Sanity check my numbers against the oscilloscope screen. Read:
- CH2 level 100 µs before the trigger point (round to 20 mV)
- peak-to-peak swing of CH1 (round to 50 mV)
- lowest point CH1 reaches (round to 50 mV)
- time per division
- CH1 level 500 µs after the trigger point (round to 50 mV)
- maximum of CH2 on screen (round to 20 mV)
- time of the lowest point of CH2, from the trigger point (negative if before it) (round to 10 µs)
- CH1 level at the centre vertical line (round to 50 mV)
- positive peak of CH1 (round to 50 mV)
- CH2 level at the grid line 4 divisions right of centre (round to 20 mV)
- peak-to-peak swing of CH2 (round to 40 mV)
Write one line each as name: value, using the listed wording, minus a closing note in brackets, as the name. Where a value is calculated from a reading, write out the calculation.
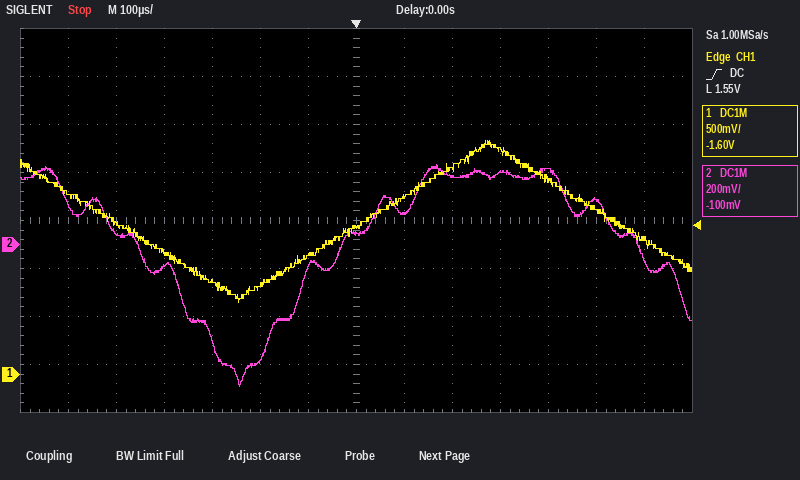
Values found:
CH2 level 100 µs before the trigger point: -100 mV
peak-to-peak swing of CH1: 2.45 V − (750 mV) = 1.70 V
lowest point CH1 reaches: 750 mV
time per division: 100 µs
CH1 level 500 µs after the trigger point: 1.70 V
maximum of CH2 on screen: 340 mV
time of the lowest point of CH2, from the trigger point (negative if before it): -240 µs
CH1 level at the centre vertical line: 1.55 V
positive peak of CH1: 2.45 V
CH2 level at the grid line 4 divisions right of centre: 320 mV
peak-to-peak swing of CH2: 920 mV
